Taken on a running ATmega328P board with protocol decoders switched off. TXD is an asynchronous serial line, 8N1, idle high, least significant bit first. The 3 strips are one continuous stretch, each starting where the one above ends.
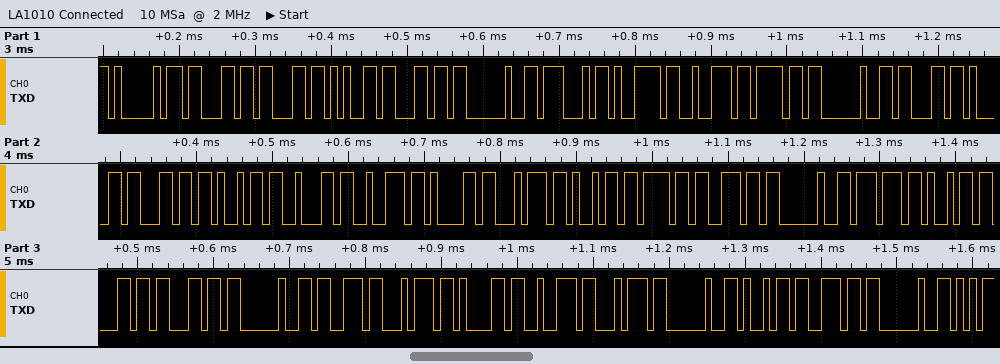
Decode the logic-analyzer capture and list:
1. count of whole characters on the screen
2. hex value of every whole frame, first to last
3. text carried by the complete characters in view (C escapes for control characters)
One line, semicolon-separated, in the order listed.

37; 41 63 63 65 6C 20 47 79 72 6F 20 63 61 6C 69 62 72 61 74 69 6F 6E 20 77 69 6C 6C 20 73 74 61 72 74 20 69 6E 20; "Accel Gyro calibration will start in "
